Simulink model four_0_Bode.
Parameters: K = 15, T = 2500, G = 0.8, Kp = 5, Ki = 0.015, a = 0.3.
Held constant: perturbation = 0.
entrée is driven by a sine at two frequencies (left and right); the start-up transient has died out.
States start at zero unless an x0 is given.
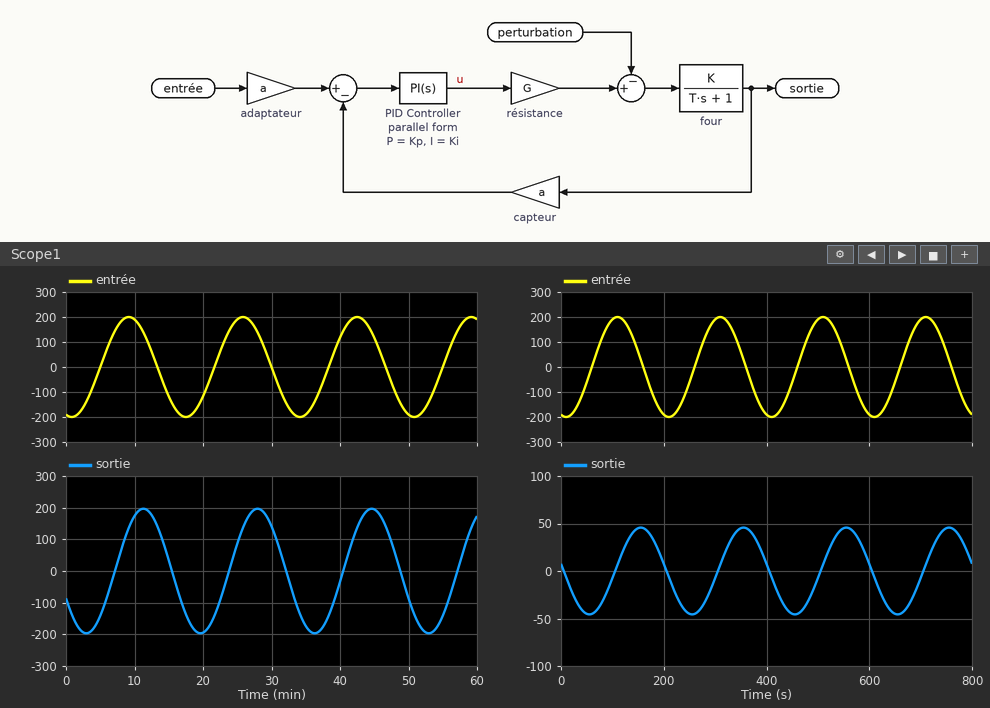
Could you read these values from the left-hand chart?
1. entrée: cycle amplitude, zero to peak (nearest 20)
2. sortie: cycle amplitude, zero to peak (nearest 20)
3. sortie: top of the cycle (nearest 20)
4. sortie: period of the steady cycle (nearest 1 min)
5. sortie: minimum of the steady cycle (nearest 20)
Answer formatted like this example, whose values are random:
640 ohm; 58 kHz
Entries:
200; 200; 200; 17 min; -200
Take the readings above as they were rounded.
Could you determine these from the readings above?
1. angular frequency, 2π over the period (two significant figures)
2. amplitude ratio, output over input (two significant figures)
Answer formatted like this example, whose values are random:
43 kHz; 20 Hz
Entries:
0.37 rad/min; 1.0
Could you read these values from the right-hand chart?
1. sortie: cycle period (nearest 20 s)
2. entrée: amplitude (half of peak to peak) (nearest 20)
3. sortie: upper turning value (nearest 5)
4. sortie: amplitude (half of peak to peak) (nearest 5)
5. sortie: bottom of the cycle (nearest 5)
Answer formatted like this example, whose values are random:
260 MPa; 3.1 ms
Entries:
200 s; 200; 45; 45; -45
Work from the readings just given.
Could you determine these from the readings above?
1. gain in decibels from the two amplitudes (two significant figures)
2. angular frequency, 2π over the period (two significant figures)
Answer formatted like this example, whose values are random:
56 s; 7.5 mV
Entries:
-13 dB; 0.031 rad/s
